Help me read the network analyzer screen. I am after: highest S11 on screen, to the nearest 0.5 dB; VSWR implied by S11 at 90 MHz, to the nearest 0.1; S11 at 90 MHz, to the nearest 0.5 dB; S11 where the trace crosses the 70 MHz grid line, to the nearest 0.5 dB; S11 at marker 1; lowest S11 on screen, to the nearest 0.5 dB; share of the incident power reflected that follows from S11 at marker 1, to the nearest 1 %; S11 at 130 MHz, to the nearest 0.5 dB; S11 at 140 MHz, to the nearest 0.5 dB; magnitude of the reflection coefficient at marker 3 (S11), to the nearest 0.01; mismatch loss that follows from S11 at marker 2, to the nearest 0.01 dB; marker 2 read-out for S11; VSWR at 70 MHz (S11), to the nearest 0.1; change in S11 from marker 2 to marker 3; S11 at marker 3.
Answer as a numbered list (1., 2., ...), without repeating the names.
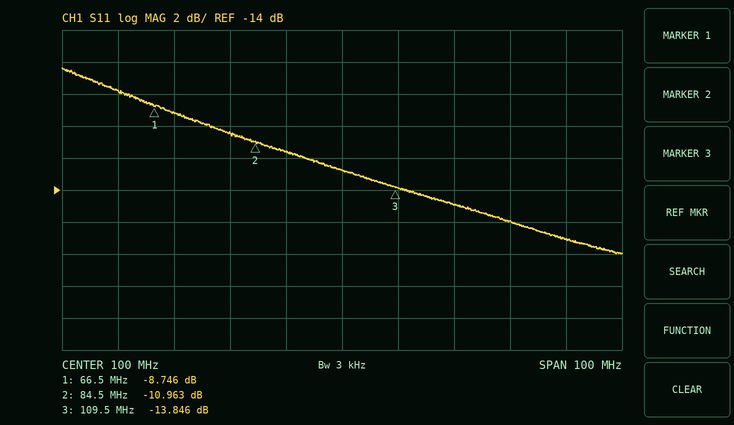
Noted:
1. -6.5 dB
2. 1.7
3. -11.5 dB
4. -9.0 dB
5. -8.746 dB
6. -18.0 dB
7. 13 %
8. -16.0 dB
9. -17.0 dB
10. 0.20
11. 0.36 dB
12. -10.963 dB
13. 2.1
14. -2.883 dB
15. -13.846 dB
